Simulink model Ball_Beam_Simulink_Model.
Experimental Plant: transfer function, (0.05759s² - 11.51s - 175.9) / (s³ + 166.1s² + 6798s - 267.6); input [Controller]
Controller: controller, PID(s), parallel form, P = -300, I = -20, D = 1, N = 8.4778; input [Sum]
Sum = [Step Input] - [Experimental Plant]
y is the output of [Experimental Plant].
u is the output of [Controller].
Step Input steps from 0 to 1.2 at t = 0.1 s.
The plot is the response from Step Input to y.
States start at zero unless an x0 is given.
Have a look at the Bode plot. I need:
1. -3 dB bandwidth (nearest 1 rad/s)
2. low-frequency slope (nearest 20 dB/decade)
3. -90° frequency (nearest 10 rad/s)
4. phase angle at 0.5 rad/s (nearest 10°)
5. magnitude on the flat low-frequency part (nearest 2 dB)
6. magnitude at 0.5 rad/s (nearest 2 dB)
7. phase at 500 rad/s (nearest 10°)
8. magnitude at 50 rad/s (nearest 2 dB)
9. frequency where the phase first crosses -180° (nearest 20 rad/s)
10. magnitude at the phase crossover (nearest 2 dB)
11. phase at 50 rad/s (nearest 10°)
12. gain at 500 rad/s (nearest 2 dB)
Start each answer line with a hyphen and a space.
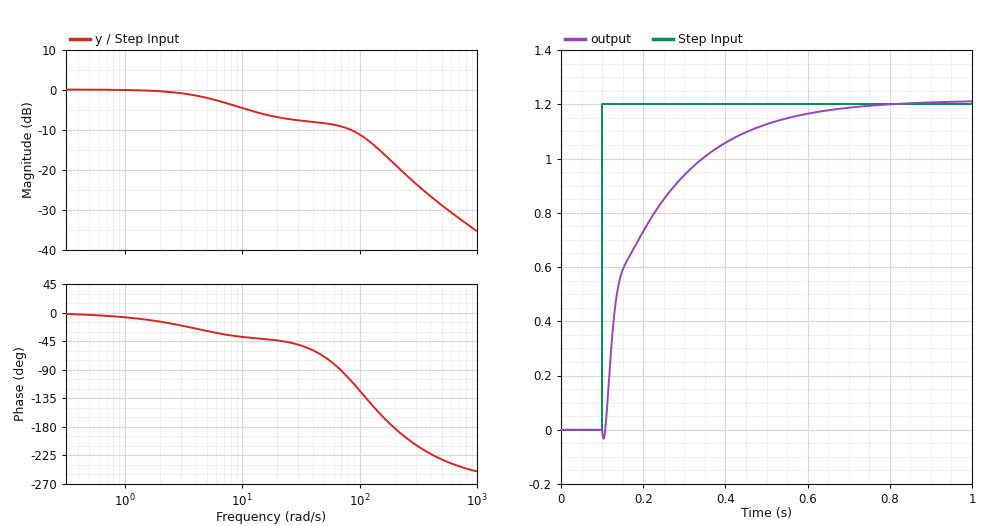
- 7 rad/s
- 0 dB/decade
- 70 rad/s
- 0°
- 0 dB
- 0 dB
- -230°
- -8 dB
- 200 rad/s
- -18 dB
- -70°
- -28 dB
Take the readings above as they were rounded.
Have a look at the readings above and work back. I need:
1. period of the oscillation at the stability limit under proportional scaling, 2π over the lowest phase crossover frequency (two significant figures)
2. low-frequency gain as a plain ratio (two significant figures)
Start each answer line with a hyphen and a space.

- 0.031 s
- 1.0
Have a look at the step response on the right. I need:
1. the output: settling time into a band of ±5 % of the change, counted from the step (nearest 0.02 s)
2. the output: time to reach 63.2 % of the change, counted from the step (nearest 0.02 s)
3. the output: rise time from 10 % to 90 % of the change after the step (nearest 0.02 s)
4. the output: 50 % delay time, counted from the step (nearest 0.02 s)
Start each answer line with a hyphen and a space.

- 0.46 s
- 0.12 s
- 0.32 s
- 0.06 s
